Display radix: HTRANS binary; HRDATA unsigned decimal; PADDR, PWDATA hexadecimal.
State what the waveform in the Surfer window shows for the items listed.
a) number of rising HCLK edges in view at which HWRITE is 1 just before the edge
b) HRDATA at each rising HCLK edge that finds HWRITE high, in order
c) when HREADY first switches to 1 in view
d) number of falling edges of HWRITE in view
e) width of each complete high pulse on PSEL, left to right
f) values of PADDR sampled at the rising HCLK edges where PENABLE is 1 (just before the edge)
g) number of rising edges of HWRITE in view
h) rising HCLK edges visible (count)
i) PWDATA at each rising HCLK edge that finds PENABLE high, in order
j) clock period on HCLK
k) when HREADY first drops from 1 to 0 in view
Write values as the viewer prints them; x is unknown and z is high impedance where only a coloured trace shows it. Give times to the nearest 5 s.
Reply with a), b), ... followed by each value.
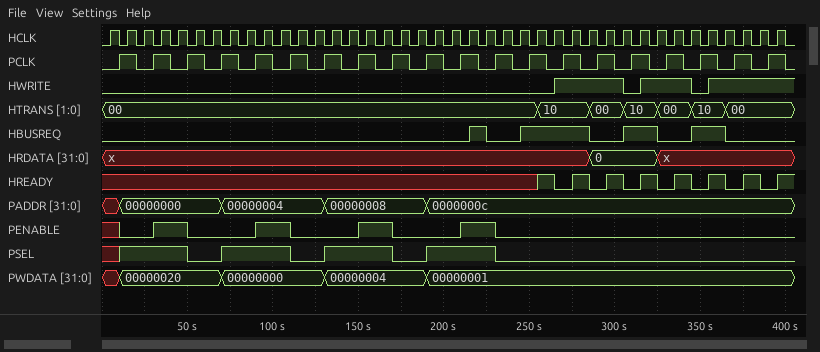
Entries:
a) 11
b) x, x, 0, 0, 0, x, x, x, x, x, x
c) 255 s
d) 2
e) 40 s, 40 s, 40 s
f) 00000000, 00000000, 00000004, 00000004, 00000008, 00000008, 0000000c, 0000000c
g) 3
h) 40
i) 00000020, 00000020, 00000000, 00000000, 00000004, 00000004, 00000001, 00000001
j) 10 s
k) 265 s
